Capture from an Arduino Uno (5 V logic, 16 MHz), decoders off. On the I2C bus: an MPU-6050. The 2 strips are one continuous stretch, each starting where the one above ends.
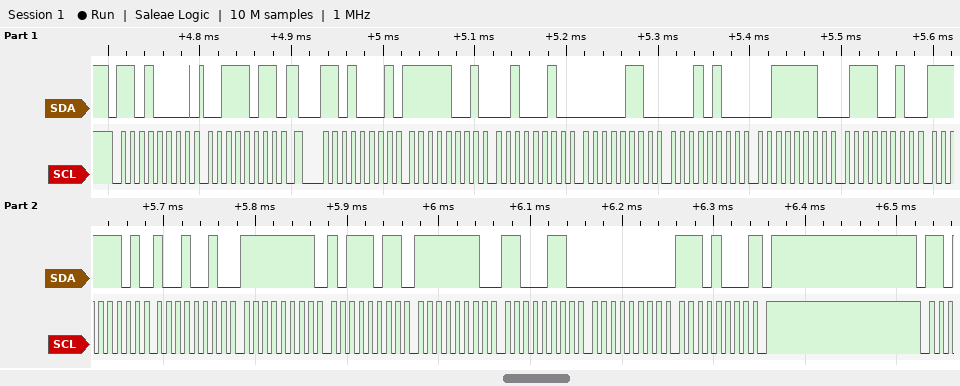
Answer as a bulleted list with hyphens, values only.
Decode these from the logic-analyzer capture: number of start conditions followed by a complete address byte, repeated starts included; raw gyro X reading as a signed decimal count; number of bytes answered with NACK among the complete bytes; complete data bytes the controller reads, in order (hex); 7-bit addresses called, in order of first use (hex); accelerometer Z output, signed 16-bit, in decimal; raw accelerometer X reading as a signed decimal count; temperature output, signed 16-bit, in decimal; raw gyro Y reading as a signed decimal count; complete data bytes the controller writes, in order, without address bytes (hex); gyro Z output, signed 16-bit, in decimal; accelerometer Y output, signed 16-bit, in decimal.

- 2
- -69
- 1
- F9 22 06 14 3E 72 FD 92 FF BB FE C6 00 E8
- 0x68
- 15986
- -1758
- -622
- -314
- 3B
- 232
- 1556
